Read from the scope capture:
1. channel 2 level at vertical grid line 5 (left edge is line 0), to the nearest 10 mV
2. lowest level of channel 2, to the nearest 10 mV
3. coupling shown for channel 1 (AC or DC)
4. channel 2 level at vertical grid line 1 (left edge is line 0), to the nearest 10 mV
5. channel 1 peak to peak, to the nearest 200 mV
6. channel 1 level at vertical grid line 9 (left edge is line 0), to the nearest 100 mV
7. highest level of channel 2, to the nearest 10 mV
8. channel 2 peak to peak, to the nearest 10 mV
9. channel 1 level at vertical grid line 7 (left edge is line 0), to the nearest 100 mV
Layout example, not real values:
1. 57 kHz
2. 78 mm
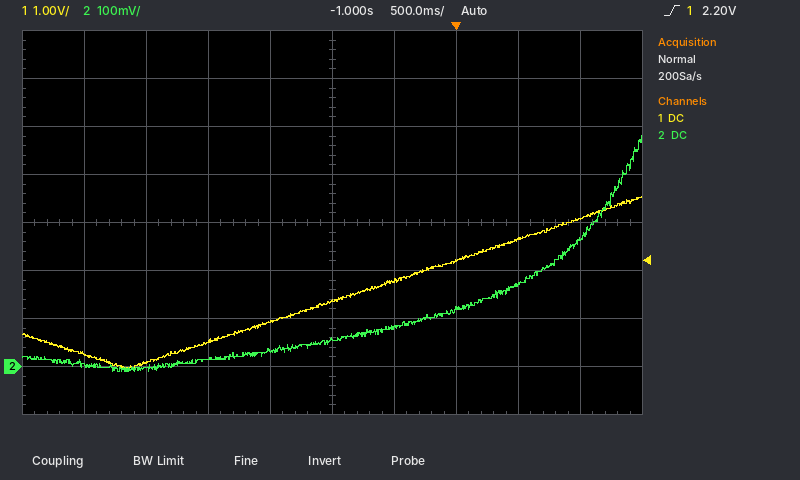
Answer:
1. 60 mV
2. -10 mV
3. DC
4. 0 mV
5. 3.6 V
6. 3.1 V
7. 480 mV
8. 490 mV
9. 2.2 V
